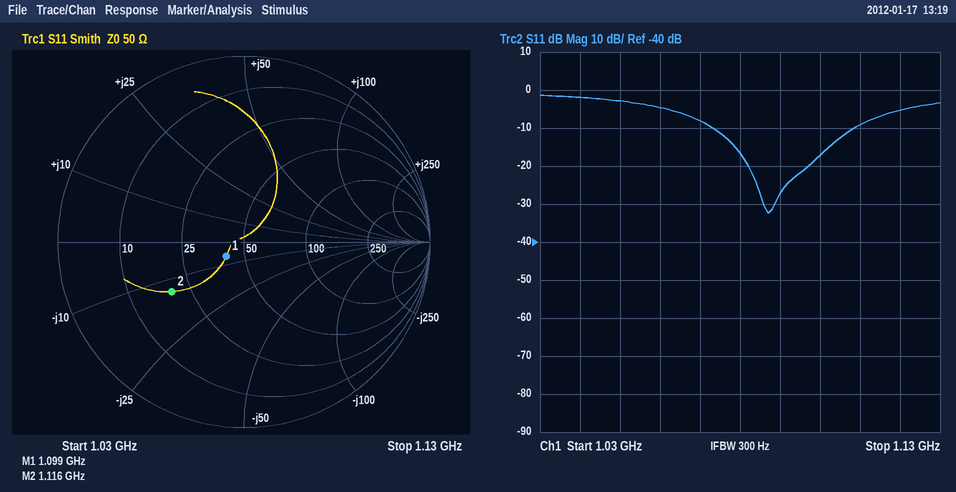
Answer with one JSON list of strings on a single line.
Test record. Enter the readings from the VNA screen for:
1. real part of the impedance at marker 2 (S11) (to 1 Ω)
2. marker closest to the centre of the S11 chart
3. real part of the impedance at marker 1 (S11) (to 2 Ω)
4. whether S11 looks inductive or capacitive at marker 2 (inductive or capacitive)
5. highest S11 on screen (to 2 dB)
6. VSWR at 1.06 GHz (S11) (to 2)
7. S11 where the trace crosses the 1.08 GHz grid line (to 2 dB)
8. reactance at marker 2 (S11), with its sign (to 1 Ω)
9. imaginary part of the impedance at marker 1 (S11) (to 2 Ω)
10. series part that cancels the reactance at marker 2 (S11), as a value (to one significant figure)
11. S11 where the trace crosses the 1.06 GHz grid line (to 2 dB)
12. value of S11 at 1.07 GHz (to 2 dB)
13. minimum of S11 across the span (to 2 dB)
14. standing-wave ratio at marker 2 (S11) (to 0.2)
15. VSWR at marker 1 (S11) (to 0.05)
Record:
["19 Ω", "marker 1", "40 Ω", "capacitive", "-2 dB", "4", "-16 dB", "-13 Ω", "-6 Ω", "2 nH", "-4 dB", "-8 dB", "-32 dB", "2.8", "1.30"]
